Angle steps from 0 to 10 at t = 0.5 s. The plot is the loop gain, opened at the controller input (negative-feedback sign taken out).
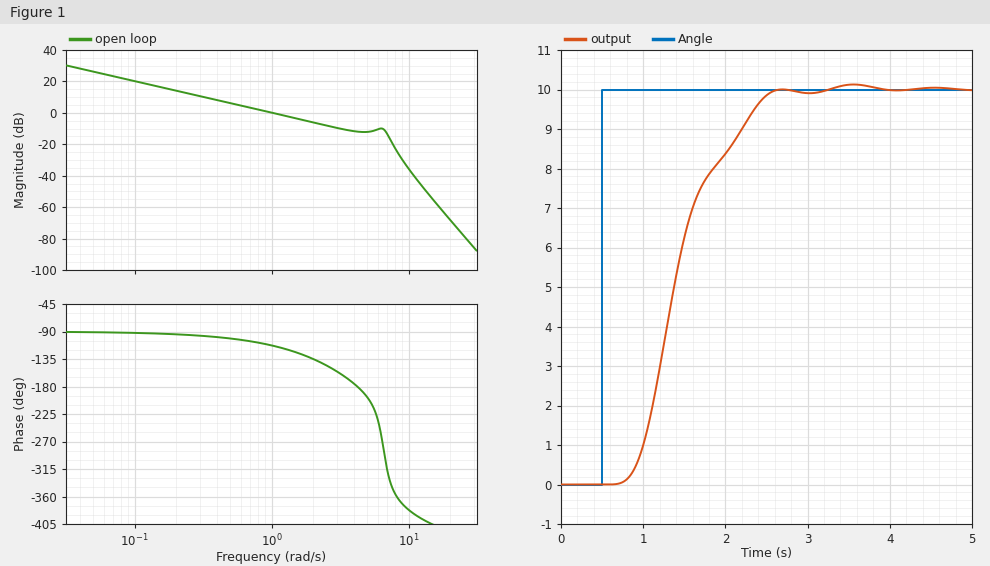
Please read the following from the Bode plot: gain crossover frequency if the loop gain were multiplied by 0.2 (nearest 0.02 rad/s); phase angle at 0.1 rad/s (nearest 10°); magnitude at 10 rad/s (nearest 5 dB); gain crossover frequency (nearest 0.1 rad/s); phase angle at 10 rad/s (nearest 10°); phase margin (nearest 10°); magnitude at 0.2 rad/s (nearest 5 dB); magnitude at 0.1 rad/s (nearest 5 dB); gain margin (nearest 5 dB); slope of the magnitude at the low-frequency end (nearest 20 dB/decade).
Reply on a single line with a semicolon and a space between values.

0.20 rad/s; -90°; -35 dB; 1.0 rad/s; -380°; 70°; 15 dB; 20 dB; 10 dB; -20 dB/decade
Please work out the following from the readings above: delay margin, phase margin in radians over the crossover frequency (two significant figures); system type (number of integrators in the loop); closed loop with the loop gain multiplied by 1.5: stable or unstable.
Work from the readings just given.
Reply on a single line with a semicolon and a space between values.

1.2 s; 1; stable
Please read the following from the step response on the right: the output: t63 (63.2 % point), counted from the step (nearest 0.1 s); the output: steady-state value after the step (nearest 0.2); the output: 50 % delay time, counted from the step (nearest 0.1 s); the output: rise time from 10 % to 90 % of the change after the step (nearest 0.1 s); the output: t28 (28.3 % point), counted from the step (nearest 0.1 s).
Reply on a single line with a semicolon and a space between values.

1.0 s; 10.0; 0.9 s; 1.2 s; 0.7 s
